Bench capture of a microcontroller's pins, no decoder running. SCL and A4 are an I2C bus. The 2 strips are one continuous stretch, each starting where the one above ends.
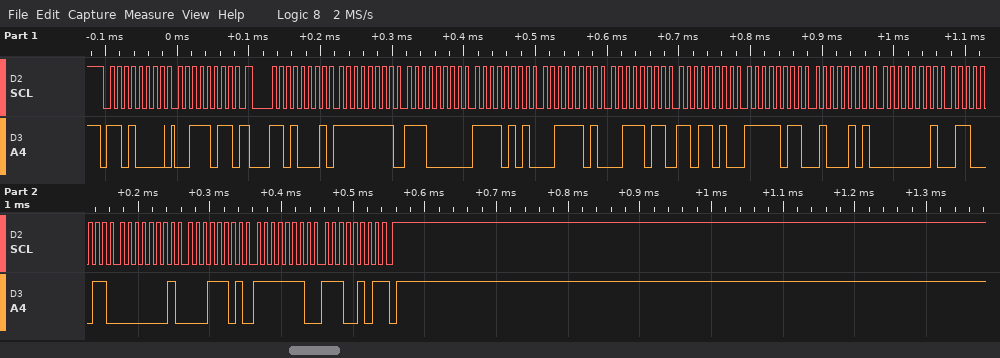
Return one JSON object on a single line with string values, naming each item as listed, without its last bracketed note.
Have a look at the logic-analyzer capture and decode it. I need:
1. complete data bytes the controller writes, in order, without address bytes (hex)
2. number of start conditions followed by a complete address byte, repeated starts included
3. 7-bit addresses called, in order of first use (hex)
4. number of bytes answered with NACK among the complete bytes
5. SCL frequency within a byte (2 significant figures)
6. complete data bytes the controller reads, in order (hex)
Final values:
{"complete data bytes the controller writes, in order, without address bytes": "3B", "number of start conditions followed by a complete address byte, repeated starts included": "2", "7-bit addresses called, in order of first use": "0x68", "number of bytes answered with NACK among the complete bytes": "1", "SCL frequency within a byte": "100 kHz", "complete data bytes the controller reads, in order": "FF E0 F5 3D 3B DA FB 45 01 63 01 1D FE E5"}
